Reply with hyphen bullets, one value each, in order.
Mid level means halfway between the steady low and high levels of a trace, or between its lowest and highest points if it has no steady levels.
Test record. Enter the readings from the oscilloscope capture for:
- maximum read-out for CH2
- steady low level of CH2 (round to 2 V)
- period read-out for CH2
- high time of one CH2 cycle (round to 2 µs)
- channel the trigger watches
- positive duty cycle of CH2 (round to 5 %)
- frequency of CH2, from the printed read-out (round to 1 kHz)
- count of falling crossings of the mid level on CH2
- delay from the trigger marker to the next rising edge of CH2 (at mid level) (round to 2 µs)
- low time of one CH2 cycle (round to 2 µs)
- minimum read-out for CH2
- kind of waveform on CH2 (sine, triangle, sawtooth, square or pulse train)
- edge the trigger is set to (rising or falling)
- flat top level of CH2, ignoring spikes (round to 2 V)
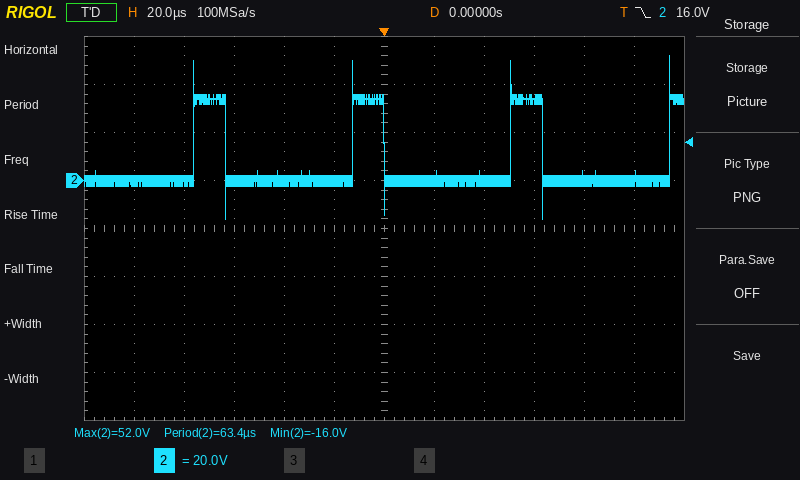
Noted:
- 52.0 V
- 0 V
- 63.4 µs
- 12 µs
- CH2
- 20 %
- 16 kHz
- 3
- 50 µs
- 50 µs
- -16.0 V
- pulse train
- falling
- 34 V
